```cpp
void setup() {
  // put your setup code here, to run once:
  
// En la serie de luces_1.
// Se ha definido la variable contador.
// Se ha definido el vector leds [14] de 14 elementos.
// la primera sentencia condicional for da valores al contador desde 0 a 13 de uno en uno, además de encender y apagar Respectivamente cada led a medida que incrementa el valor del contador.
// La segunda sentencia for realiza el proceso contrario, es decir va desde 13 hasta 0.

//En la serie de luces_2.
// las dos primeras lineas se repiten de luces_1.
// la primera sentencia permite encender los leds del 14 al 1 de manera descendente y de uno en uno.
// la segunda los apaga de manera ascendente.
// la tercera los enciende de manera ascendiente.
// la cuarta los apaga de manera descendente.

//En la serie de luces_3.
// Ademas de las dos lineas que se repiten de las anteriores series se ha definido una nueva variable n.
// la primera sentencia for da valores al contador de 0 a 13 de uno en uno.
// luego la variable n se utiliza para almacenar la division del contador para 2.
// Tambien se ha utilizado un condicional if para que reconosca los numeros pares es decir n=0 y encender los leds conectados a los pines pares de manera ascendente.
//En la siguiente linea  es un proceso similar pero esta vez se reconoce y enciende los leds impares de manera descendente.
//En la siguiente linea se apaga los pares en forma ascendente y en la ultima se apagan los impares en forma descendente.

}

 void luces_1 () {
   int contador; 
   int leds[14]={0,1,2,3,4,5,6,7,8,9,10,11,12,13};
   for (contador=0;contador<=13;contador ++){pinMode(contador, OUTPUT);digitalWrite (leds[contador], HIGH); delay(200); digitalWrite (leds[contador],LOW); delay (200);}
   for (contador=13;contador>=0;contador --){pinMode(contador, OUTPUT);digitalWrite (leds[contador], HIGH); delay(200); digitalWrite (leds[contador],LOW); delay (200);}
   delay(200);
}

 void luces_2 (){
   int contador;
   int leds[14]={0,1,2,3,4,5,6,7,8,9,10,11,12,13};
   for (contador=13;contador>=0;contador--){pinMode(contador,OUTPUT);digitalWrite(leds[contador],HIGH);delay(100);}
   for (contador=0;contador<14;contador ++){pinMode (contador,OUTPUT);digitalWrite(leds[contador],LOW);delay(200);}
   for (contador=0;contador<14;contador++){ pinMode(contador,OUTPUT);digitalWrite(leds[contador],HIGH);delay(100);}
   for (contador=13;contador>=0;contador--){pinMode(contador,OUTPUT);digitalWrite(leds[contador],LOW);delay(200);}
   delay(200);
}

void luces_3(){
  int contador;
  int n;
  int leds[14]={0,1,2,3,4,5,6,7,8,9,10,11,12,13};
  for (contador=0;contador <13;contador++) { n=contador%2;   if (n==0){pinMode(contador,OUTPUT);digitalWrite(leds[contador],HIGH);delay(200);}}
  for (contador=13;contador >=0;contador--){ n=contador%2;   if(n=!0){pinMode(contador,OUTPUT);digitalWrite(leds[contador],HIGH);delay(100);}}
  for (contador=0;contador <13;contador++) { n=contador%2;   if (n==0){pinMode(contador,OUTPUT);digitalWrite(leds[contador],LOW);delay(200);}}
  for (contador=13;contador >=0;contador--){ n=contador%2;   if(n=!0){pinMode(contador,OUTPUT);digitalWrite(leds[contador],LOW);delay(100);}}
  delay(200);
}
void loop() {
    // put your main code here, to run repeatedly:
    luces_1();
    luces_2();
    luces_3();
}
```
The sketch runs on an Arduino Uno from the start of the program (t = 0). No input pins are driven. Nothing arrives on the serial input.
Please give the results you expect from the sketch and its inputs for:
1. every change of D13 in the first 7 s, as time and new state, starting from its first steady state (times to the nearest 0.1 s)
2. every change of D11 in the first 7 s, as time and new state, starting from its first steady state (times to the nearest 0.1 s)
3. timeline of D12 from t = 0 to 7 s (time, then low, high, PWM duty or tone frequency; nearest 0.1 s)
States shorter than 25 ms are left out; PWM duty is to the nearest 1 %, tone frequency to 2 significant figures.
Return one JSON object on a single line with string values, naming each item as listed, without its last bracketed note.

{"every change of D13 in the first 7 s, as time and new state, starting from its first steady state": "5.2 s high; 5.4 s low; 5.6 s high; 5.8 s low", "every change of D11 in the first 7 s, as time and new state, starting from its first steady state": "4.4 s high; 4.6 s low; 6.4 s high; 6.6 s low", "timeline of D12 from t = 0 to 7 s": "4.8 s high; 5 s low; 6 s high; 6.2 s low"}
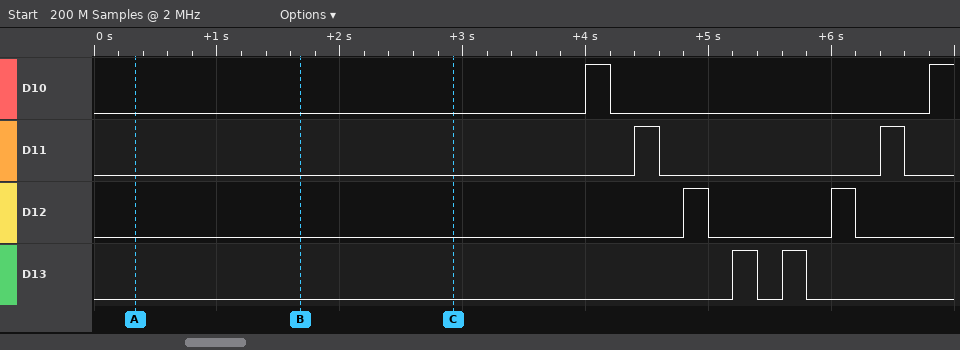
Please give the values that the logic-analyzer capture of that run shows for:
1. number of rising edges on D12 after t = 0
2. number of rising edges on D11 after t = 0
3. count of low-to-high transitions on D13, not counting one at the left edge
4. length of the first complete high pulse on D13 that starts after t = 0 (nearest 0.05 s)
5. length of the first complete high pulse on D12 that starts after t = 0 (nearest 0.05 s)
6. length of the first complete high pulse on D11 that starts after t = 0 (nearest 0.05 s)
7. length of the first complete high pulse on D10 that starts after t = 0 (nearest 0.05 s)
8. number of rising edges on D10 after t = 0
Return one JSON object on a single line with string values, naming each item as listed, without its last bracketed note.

{"number of rising edges on D12 after t = 0": "2", "number of rising edges on D11 after t = 0": "2", "count of low-to-high transitions on D13, not counting one at the left edge": "2", "length of the first complete high pulse on D13 that starts after t = 0": "0.20 s", "length of the first complete high pulse on D12 that starts after t = 0": "0.20 s", "length of the first complete high pulse on D11 that starts after t = 0": "0.20 s", "length of the first complete high pulse on D10 that starts after t = 0": "0.20 s", "number of rising edges on D10 after t = 0": "2"}
